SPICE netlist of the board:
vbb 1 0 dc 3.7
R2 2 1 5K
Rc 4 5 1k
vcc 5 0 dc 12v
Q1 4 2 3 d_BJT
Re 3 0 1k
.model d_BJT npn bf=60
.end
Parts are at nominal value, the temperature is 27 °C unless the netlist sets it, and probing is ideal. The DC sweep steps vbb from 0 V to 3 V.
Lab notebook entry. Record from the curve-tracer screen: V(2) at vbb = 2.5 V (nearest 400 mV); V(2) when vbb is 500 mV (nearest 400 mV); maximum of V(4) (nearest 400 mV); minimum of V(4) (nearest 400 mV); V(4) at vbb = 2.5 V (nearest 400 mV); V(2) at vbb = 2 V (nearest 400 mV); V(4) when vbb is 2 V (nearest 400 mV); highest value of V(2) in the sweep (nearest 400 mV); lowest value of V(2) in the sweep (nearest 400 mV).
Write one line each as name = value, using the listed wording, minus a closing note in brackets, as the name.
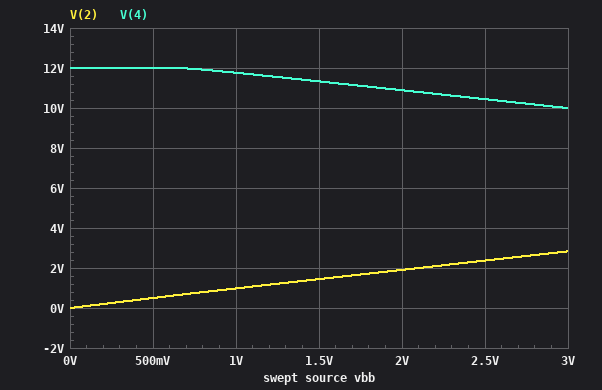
V(2) at vbb = 2.5 V = 2.4 V
V(2) when vbb is 500 mV = 400 mV
maximum of V(4) = 12.0 V
minimum of V(4) = 10.0 V
V(4) at vbb = 2.5 V = 10.4 V
V(2) at vbb = 2 V = 2.0 V
V(4) when vbb is 2 V = 10.8 V
highest value of V(2) in the sweep = 2.8 V
lowest value of V(2) in the sweep = 0 V
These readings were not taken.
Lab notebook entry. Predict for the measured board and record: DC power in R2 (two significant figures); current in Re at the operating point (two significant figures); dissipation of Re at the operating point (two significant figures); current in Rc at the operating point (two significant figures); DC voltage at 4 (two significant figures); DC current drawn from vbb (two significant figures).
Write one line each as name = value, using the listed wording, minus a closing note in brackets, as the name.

DC power in R2 = 9.7 µW
current in Re at the operating point = 2.7 mA
dissipation of Re at the operating point = 7.2 mW
current in Rc at the operating point = 2.6 mA
DC voltage at 4 = 9.4 V
DC current drawn from vbb = 44 µA
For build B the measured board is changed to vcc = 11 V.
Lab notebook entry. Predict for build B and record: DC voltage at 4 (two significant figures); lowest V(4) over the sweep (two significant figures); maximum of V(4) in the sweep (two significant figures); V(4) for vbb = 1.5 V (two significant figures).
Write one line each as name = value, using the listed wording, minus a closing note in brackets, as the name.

DC voltage at 4 = 8.4 V
lowest V(4) over the sweep = 9.0 V
maximum of V(4) in the sweep = 11 V
V(4) for vbb = 1.5 V = 10 V
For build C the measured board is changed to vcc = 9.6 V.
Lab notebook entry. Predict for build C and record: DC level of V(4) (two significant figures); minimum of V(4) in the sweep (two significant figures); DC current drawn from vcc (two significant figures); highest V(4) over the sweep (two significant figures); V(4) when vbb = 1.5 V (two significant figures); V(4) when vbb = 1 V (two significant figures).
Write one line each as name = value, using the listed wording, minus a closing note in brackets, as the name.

DC level of V(4) = 7.0 V
minimum of V(4) in the sweep = 7.6 V
DC current drawn from vcc = 2.6 mA
highest V(4) over the sweep = 9.6 V
V(4) when vbb = 1.5 V = 8.9 V
V(4) when vbb = 1 V = 9.4 V
